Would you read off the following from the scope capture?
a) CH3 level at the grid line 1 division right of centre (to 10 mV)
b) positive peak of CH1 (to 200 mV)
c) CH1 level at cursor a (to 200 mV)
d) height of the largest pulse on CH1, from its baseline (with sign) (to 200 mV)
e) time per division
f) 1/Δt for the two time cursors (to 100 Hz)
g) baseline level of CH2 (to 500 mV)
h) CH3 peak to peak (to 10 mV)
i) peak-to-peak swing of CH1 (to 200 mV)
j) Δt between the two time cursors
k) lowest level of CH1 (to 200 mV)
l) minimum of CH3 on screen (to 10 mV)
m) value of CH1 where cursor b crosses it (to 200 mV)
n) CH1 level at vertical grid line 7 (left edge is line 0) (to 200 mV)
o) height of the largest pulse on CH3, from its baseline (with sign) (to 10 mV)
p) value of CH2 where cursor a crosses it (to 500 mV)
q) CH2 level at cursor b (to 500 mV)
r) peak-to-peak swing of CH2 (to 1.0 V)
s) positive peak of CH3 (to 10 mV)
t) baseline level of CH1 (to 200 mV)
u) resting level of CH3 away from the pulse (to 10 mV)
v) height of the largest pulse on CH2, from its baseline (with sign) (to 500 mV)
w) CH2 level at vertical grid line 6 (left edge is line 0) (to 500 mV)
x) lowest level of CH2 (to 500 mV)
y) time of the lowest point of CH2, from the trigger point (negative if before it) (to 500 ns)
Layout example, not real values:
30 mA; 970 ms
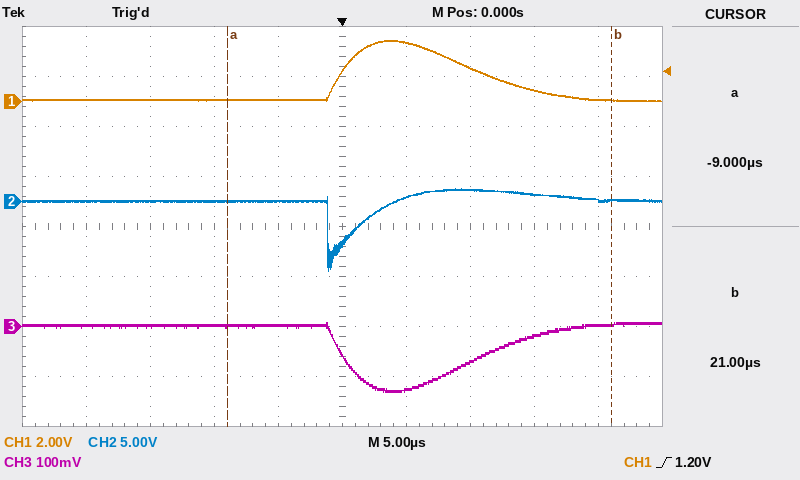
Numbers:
-130 mV; 2.4 V; 0.0 V; +2.4 V; 5 µs; 33.3 kHz; 0.0 V; 140 mV; 2.4 V; 30.0 µs; 0.0 V; -130 mV; 0.0 V; 1.4 V; -130 mV; 0.0 V; 0.0 V; 8.0 V; 10 mV; 0.0 V; 0 mV; -7.0 V; 500 mV; -7.0 V; -1.0 µs
